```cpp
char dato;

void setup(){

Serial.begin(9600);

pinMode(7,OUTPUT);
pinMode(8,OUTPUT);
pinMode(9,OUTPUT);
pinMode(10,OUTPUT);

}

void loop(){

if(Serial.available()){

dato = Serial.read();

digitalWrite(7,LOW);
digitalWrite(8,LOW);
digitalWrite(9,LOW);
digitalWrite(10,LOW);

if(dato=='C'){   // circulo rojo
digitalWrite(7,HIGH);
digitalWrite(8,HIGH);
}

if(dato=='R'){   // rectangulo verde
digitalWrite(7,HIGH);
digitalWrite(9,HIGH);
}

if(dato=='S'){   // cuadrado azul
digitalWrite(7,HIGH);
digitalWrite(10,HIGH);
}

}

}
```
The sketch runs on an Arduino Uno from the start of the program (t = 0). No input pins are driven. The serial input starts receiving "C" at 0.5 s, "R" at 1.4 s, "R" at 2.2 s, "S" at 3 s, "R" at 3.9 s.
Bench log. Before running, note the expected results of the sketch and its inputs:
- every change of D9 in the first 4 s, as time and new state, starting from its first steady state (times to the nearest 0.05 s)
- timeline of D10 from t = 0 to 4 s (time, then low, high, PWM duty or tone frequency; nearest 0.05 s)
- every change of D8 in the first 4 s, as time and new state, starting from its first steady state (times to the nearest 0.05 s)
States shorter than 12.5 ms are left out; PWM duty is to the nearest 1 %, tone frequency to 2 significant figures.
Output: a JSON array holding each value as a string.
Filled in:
["0 s low; 1.4 s high; 3 s low; 3.9 s high", "0 s low; 3 s high; 3.9 s low", "0 s low; 0.5 s high; 1.4 s low"]
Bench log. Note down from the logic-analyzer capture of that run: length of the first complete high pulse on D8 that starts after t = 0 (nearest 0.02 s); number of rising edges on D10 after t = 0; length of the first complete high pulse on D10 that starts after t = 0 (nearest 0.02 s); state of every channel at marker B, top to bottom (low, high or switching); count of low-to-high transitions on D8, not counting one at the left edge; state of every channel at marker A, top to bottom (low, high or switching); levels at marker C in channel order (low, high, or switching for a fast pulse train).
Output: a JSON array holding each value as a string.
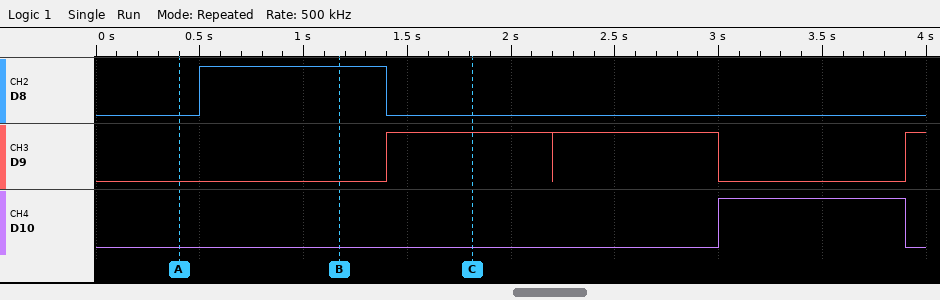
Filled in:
["0.90 s", "1", "0.90 s", "D8 high, D9 low, D10 low", "1", "D8 low, D9 low, D10 low", "D8 low, D9 high, D10 low"]
